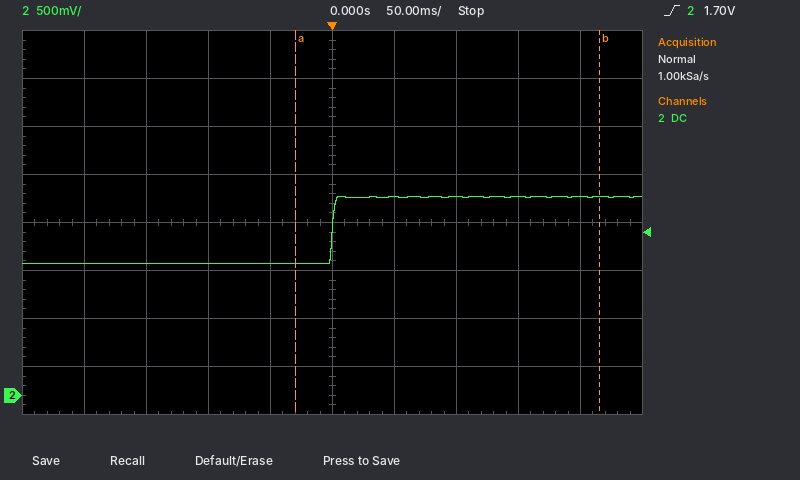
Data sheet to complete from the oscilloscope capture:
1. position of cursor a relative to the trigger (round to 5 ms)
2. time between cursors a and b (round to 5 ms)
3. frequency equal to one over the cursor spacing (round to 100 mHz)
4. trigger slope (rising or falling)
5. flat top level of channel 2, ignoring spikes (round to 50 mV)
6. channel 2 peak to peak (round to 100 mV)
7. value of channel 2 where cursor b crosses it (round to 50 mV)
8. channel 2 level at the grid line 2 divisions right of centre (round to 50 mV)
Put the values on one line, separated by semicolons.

-30 ms; 245 ms; 4.1 Hz; rising; 2.05 V; 700 mV; 2.05 V; 2.05 V
